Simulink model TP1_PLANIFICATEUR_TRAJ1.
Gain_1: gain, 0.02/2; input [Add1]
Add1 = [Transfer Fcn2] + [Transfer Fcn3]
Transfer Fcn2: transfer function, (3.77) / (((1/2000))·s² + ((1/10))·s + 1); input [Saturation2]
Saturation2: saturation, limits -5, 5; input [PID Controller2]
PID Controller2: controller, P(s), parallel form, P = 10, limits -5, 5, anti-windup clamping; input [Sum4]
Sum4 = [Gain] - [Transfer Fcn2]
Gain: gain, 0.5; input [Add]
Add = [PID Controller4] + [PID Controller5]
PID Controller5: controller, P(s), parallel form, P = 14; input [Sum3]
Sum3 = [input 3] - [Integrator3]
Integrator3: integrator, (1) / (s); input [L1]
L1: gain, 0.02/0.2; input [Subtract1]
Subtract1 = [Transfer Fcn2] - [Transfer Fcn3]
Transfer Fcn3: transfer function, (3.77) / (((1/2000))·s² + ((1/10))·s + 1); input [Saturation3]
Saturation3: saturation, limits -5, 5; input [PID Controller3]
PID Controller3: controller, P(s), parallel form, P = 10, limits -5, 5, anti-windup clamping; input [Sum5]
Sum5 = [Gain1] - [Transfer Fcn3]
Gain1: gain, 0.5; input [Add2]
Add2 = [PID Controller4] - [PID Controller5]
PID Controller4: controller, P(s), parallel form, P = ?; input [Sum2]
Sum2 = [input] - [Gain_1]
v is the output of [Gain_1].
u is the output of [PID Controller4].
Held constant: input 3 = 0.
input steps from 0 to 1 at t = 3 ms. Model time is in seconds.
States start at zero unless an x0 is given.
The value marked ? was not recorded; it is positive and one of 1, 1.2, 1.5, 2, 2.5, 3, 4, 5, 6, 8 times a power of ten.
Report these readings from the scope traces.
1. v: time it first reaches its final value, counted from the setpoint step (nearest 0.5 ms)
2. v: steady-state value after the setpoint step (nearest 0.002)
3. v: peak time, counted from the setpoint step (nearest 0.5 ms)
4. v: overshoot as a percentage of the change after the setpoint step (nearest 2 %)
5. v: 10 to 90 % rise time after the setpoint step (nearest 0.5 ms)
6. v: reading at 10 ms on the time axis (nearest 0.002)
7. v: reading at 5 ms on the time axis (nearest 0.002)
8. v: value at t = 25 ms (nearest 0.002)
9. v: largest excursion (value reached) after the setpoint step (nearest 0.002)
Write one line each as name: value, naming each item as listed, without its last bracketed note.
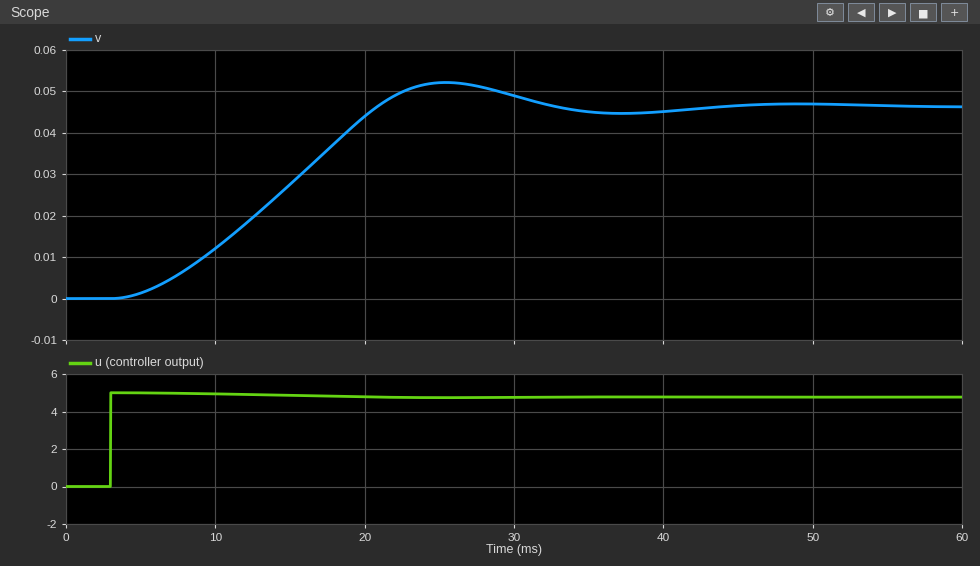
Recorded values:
v: time it first reaches its final value, counted from the setpoint step: 18.0 ms
v: steady-state value after the setpoint step: 0.046
v: peak time, counted from the setpoint step: 22.5 ms
v: overshoot as a percentage of the change after the setpoint step: 12 %
v: 10 to 90 % rise time after the setpoint step: 12.5 ms
v: reading at 10 ms on the time axis: 0.012
v: reading at 5 ms on the time axis: 0.002
v: value at t = 25 ms: 0.052
v: largest excursion (value reached) after the setpoint step: 0.052
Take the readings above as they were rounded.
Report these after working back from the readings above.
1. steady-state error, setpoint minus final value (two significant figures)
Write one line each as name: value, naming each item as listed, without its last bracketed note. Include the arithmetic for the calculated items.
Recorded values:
steady-state error, setpoint minus final value: 1 - 0.046 = 0.95
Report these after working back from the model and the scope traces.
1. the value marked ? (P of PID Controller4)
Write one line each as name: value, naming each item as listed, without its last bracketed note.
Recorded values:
the value marked ?: 5
